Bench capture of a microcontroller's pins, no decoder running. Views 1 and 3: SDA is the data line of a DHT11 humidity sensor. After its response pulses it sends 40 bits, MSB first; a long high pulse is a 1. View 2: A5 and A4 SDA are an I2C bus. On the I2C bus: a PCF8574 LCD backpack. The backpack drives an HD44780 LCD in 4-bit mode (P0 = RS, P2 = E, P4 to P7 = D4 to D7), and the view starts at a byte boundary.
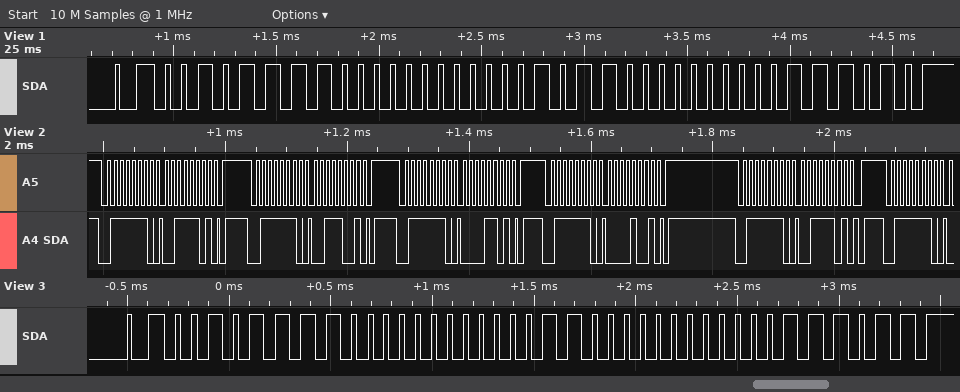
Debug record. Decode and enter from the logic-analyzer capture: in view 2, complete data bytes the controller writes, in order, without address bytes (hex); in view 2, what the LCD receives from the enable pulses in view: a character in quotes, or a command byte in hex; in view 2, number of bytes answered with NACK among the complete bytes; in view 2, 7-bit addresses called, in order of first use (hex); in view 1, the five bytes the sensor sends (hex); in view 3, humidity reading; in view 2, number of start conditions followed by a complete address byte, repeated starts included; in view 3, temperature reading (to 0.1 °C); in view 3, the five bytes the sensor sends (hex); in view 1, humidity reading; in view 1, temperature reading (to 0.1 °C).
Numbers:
3D 39 0D 09 3D
'0'
0
0x3F
2F 00 0B 00 3A
47 %
6
12.0 °C
2F 00 0C 00 3B
47 %
11.0 °C
